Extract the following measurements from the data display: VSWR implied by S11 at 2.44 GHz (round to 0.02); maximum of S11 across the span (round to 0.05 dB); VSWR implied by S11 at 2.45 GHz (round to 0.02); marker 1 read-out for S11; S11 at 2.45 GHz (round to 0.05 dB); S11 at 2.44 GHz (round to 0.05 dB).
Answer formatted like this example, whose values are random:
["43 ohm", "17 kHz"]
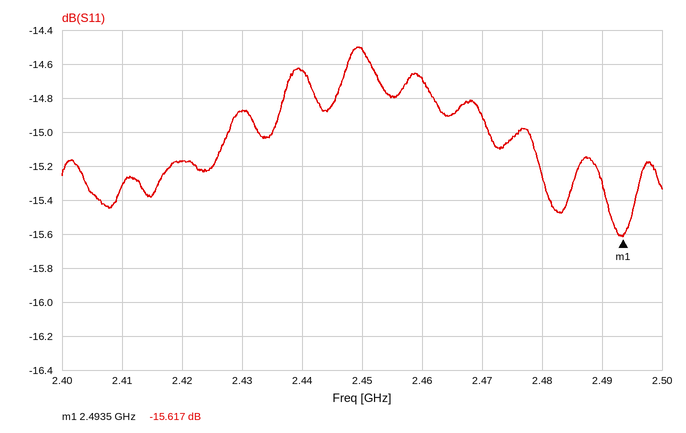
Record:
["1.46", "-14.50 dB", "1.46", "-15.617 dB", "-14.50 dB", "-14.65 dB"]
